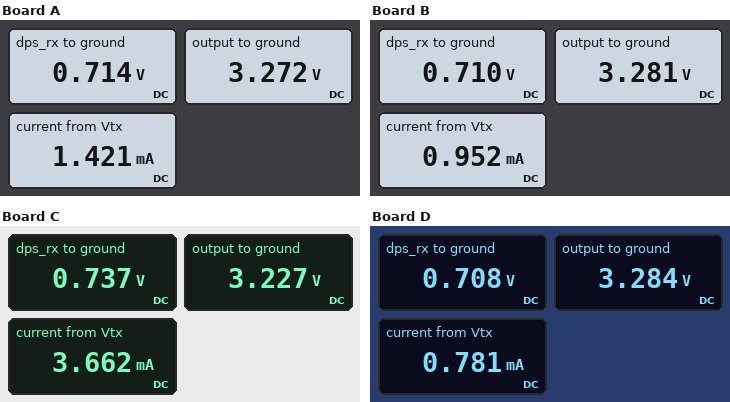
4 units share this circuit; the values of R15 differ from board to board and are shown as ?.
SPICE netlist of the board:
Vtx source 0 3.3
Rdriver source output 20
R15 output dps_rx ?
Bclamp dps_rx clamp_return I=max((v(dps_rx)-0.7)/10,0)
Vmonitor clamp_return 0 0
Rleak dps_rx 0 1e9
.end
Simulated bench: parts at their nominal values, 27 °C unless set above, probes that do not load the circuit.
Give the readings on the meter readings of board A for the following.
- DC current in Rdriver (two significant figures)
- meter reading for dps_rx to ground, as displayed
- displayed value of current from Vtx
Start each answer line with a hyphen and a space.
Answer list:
- 1.4 mA
- 0.714 V
- 1.421 mA
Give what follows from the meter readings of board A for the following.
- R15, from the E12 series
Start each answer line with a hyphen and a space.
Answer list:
- 1.8 kΩ
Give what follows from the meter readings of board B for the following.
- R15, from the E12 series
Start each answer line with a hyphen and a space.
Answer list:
- 2.7 kΩ
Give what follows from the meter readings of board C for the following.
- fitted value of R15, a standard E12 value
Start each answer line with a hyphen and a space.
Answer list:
- 680 Ω
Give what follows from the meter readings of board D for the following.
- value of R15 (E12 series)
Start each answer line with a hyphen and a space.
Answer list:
- 3.3 kΩ
